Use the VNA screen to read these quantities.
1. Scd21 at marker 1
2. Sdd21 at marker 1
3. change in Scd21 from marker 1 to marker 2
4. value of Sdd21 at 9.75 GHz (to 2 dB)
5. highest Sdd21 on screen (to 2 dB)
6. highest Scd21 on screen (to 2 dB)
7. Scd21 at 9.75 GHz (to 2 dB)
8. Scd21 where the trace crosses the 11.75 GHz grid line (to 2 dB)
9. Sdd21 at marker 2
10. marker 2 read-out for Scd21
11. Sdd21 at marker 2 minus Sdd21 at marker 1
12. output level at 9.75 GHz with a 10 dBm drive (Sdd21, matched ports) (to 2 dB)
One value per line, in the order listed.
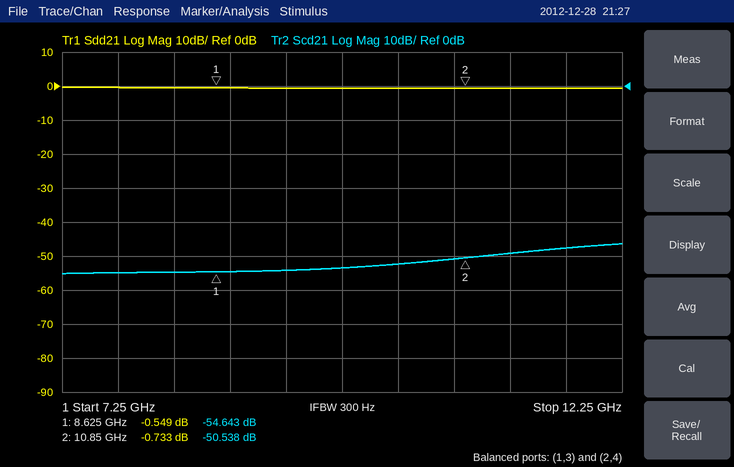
-54.643 dB
-0.549 dB
4.105 dB
0 dB
0 dB
-46 dB
-54 dB
-48 dB
-0.733 dB
-50.538 dB
-0.184 dB
10 dBm
